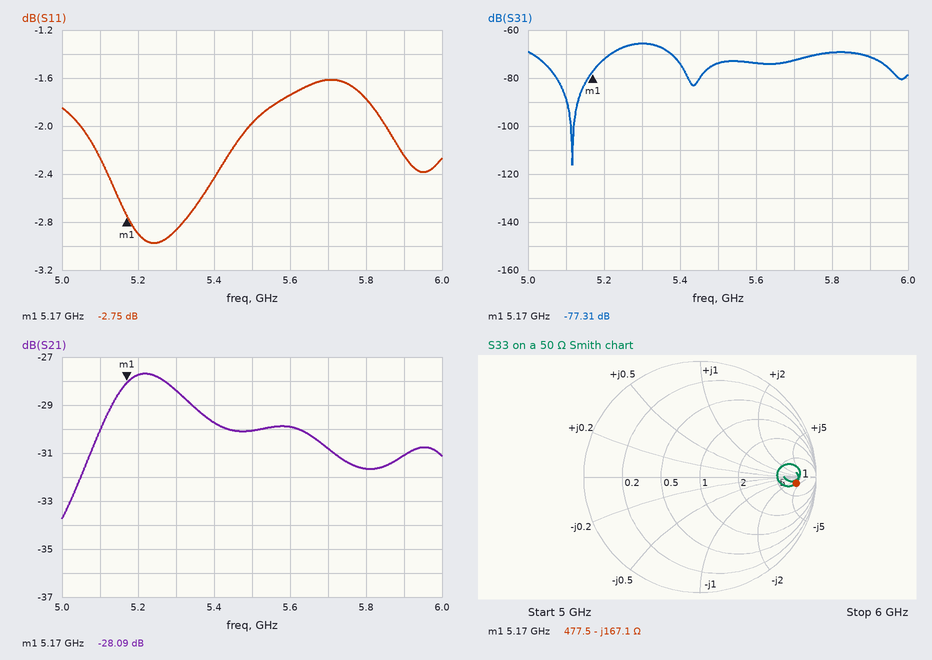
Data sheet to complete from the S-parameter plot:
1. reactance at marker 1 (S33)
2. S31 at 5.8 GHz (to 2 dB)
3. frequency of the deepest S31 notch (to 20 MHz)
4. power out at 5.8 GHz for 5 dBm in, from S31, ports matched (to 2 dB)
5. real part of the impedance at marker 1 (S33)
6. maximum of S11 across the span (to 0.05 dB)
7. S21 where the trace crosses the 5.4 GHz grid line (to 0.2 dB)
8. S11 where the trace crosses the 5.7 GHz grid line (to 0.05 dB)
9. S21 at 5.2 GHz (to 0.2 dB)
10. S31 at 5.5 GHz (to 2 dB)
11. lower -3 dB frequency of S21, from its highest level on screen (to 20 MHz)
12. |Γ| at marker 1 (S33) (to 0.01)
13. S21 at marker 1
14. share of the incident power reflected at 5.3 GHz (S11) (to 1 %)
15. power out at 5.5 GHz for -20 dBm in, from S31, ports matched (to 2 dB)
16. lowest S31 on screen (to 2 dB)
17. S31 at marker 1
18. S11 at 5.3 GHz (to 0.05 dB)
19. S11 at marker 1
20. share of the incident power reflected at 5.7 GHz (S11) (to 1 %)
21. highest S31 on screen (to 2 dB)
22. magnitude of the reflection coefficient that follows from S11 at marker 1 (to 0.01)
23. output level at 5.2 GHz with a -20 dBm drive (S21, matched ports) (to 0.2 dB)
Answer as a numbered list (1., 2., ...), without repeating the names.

1. -167.1 Ω
2. -70 dB
3. 5.12 GHz
4. -64 dBm
5. 477.5 Ω
6. -1.60 dB
7. -29.8 dB
8. -1.60 dB
9. -27.8 dB
10. -74 dB
11. 5.08 GHz
12. 0.83
13. -28.09 dB
14. 52 %
15. -94 dBm
16. -116 dB
17. -77.31 dB
18. -2.85 dB
19. -2.75 dB
20. 69 %
21. -66 dB
22. 0.73
23. -47.8 dBm
